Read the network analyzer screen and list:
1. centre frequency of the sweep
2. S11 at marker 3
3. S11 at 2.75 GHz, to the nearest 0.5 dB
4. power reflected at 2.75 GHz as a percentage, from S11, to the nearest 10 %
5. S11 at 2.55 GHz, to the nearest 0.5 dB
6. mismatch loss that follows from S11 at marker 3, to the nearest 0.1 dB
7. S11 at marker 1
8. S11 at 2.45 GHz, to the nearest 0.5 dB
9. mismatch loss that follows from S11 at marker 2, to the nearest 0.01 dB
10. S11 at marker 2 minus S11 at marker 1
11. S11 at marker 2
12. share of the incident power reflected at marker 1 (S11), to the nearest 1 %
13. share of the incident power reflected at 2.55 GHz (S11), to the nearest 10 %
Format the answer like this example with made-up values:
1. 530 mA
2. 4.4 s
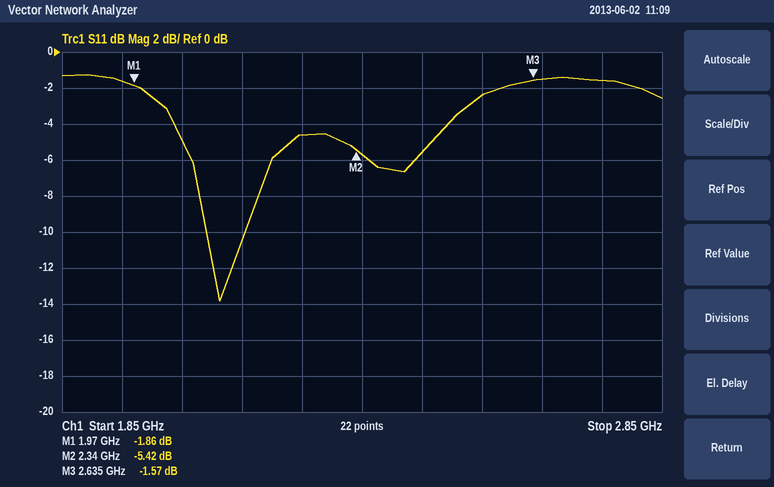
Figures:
1. 2.35 GHz
2. -1.57 dB
3. -1.5 dB
4. 70 %
5. -2.5 dB
6. 5.2 dB
7. -1.86 dB
8. -5.5 dB
9. 1.47 dB
10. -3.56 dB
11. -5.42 dB
12. 65 %
13. 60 %
